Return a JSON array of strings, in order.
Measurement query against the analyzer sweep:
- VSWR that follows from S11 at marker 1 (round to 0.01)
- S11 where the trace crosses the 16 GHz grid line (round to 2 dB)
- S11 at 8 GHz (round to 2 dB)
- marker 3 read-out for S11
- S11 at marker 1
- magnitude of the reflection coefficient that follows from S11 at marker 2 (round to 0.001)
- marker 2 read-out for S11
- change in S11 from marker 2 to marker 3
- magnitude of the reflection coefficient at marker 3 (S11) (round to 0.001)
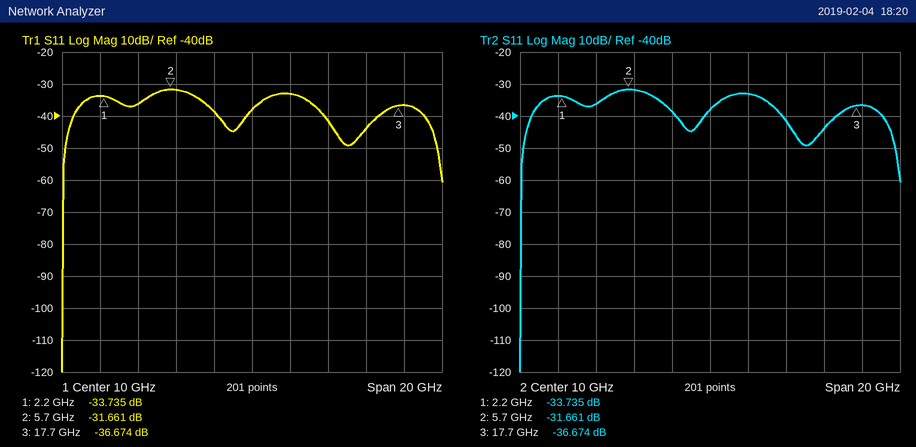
["1.04", "-44 dB", "-38 dB", "-36.674 dB", "-33.735 dB", "0.026", "-31.661 dB", "-5.013 dB", "0.015"]
